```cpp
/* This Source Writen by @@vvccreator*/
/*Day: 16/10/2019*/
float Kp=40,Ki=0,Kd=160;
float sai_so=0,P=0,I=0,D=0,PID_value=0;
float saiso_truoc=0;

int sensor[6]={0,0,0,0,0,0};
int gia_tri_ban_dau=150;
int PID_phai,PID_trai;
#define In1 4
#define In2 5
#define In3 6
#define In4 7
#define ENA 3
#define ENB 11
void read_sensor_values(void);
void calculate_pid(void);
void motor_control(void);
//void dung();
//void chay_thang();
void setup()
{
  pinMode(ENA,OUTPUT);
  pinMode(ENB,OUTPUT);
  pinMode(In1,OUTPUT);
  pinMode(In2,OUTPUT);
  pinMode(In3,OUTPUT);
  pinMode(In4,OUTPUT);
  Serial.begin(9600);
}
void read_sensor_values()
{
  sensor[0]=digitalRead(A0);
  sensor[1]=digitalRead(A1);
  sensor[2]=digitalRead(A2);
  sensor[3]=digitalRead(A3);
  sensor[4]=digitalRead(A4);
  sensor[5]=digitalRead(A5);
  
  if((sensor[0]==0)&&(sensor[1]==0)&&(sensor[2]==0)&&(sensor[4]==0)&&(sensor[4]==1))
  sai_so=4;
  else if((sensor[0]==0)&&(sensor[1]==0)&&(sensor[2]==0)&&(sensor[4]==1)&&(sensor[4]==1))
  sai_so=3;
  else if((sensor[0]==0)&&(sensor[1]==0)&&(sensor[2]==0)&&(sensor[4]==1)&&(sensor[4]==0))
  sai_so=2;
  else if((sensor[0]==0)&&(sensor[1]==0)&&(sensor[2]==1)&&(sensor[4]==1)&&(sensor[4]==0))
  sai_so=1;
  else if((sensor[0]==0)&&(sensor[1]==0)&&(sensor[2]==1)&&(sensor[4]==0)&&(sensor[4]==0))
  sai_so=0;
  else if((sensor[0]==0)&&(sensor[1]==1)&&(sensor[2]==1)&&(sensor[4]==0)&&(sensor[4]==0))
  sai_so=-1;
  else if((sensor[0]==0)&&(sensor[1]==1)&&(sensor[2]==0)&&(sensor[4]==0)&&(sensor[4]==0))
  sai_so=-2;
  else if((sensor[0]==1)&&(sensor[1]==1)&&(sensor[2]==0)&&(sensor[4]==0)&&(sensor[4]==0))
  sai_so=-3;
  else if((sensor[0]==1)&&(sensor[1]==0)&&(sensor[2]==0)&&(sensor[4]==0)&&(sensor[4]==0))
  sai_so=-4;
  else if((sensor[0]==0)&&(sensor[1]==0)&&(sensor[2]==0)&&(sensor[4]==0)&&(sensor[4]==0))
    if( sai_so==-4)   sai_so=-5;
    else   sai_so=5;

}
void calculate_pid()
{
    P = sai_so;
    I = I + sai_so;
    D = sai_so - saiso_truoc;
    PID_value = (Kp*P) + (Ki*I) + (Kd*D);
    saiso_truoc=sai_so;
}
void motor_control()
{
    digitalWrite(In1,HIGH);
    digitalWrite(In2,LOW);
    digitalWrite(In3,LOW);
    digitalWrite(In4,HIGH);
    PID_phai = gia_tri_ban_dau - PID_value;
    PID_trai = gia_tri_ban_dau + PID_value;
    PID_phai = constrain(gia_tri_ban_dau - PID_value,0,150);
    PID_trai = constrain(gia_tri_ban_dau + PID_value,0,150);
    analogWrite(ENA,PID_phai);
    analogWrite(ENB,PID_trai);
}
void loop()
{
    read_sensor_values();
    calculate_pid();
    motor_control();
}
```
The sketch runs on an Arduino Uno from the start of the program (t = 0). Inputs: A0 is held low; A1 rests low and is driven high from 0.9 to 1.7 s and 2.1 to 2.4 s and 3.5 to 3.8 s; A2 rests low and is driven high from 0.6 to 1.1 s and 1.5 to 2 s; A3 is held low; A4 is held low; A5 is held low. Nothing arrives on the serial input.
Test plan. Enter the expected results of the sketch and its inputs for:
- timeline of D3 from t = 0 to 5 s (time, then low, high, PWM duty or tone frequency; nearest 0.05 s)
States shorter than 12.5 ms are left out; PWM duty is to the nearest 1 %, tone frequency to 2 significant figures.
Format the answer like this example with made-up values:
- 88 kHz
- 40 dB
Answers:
- 0 s low; 0.6 s PWM 59 %; 2 s low; 2.1 s PWM 59 %; 2.4 s low; 3.5 s PWM 59 %; 3.8 s low
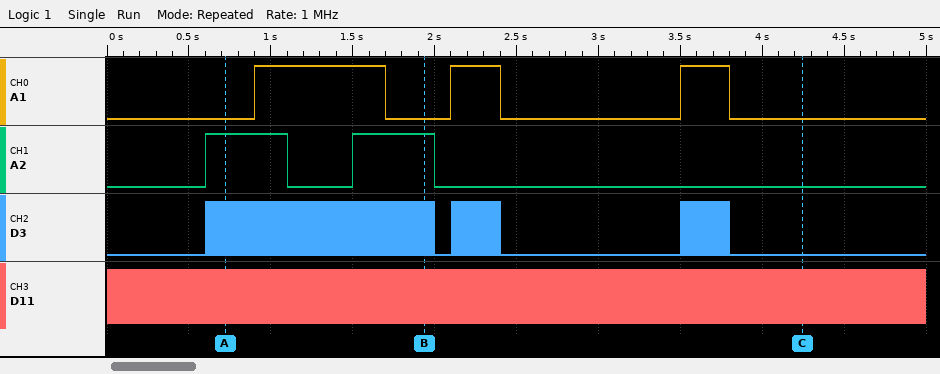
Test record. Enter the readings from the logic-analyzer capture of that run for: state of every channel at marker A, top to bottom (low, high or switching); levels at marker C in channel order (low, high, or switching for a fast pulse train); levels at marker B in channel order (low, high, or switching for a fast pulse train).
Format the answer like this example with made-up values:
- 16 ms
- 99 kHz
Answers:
- A1 low, A2 high, D3 switching, D11 switching
- A1 low, A2 low, D3 low, D11 switching
- A1 low, A2 high, D3 switching, D11 switching
